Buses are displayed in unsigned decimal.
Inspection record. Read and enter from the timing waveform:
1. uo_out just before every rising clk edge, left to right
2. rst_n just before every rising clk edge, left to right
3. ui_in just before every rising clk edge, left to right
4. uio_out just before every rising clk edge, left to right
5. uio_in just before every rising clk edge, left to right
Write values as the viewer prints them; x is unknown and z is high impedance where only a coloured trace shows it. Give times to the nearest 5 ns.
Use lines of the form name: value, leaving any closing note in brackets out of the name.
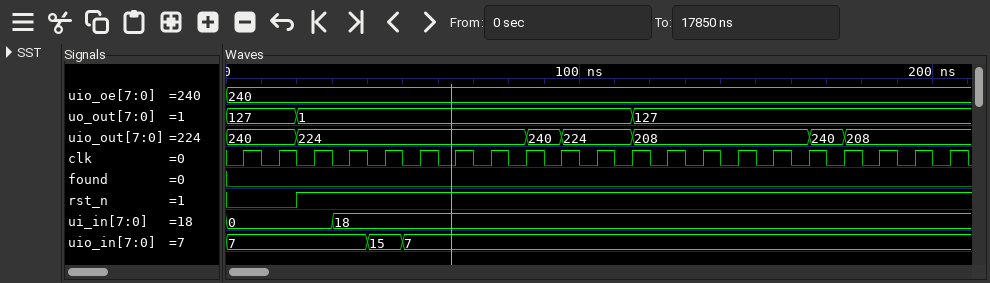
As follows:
uo_out just before every rising clk edge, left to right: 127, 127, 1, 1, 1, 1, 1, 1, 1, 1, 1, 1, 127, 127, 127, 127, 127, 127, 127, 127, 127
rst_n just before every rising clk edge, left to right: 0 0 1 1 1 1 1 1 1 1 1 1 1 1 1 1 1 1 1 1 1
ui_in just before every rising clk edge, left to right: 0, 0, 0, 18, 18, 18, 18, 18, 18, 18, 18, 18, 18, 18, 18, 18, 18, 18, 18, 18, 18
uio_out just before every rising clk edge, left to right: 240, 240, 224, 224, 224, 224, 224, 224, 224, 240, 224, 224, 208, 208, 208, 208, 208, 240, 208, 208, 208
uio_in just before every rising clk edge, left to right: 7, 7, 7, 7, 15, 7, 7, 7, 7, 7, 7, 7, 7, 7, 7, 7, 7, 7, 7, 7, 7
